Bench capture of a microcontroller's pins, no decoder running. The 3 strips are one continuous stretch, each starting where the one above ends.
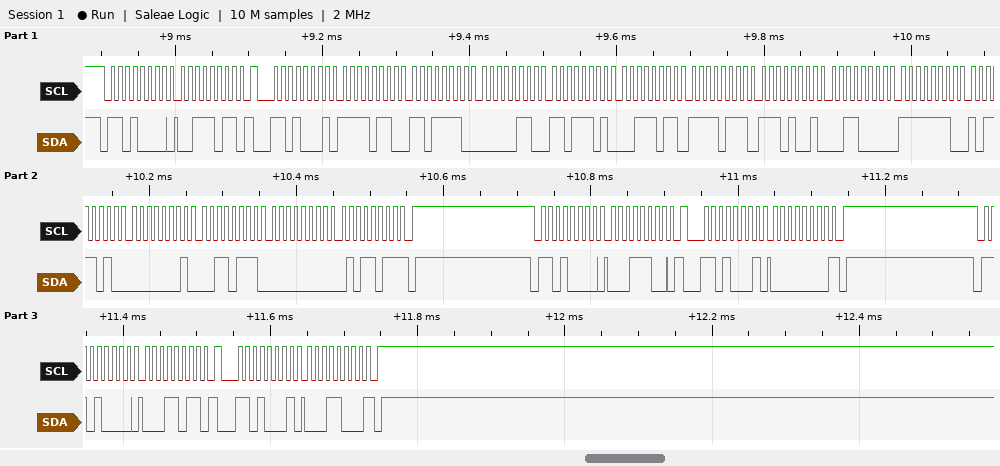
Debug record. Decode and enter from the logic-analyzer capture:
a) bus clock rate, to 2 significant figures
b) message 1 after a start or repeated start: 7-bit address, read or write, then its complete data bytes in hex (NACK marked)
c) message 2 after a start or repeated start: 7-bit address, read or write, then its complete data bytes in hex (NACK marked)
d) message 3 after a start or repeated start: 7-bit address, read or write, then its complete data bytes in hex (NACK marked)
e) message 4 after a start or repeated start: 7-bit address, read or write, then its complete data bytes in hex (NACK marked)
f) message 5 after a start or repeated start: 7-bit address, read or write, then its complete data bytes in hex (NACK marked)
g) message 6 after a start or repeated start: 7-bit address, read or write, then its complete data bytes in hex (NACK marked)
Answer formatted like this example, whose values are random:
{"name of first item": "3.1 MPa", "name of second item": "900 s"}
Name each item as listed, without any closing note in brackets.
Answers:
{"bus clock rate, to 2 significant figures": "100 kHz", "message 1 after a start or repeated start: 7-bit address, read or write, then its complete data bytes in hex": "0x68 write: 3B", "message 2 after a start or repeated start: 7-bit address, read or write, then its complete data bytes in hex": "0x68 read: F6 DE 06 DD 3B F7 E9 30 FE BA 01 37 00 5B NACK", "message 3 after a start or repeated start: 7-bit address, read or write, then its complete data bytes in hex": "0x68 write: 1C", "message 4 after a start or repeated start: 7-bit address, read or write, then its complete data bytes in hex": "0x68 read: 00 NACK", "message 5 after a start or repeated start: 7-bit address, read or write, then its complete data bytes in hex": "0x68 write: 1B", "message 6 after a start or repeated start: 7-bit address, read or write, then its complete data bytes in hex": "0x68 read: 18 NACK"}
